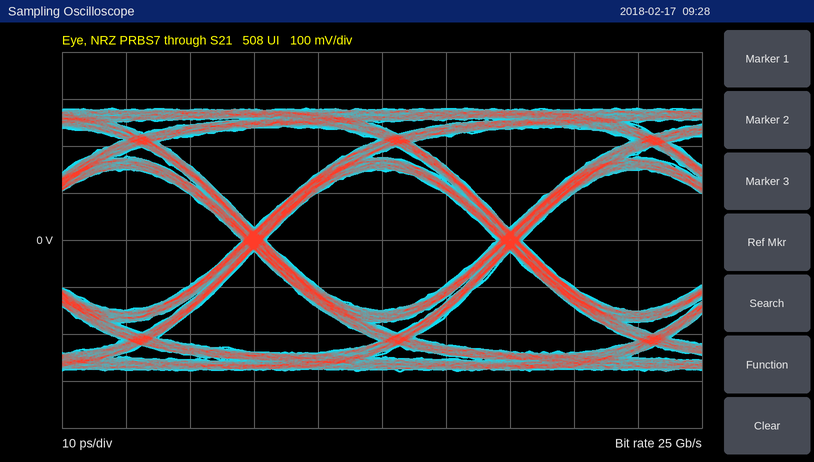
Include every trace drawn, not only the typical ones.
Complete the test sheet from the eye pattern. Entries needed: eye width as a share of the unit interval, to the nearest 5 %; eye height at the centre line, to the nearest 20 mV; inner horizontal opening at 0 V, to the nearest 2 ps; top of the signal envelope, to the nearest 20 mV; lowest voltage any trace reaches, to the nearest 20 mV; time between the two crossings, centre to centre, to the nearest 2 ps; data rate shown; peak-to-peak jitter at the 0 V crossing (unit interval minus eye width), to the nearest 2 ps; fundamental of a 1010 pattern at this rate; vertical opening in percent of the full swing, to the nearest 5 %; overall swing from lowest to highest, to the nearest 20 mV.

90 %
300 mV
36 ps
280 mV
-280 mV
40 ps
25 Gb/s
4 ps
12.5 GHz
55 %
560 mV
